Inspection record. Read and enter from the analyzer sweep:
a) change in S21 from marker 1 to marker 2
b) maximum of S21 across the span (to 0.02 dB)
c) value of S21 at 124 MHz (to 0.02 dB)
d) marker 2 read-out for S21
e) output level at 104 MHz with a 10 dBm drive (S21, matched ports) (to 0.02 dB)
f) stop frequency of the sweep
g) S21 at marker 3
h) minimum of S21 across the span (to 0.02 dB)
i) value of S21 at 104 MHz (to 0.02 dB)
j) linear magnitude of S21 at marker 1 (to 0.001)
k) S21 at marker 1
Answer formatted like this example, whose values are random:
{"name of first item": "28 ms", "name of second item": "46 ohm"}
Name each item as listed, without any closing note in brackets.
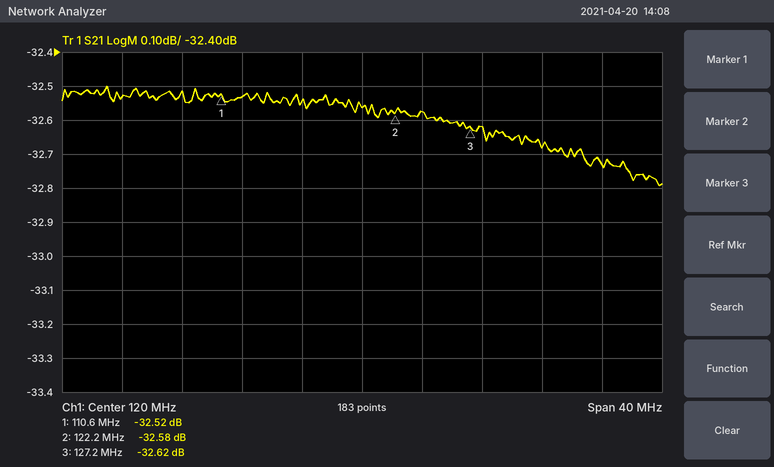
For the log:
{"change in S21 from marker 1 to marker 2": "-0.06 dB", "maximum of S21 across the span": "-32.50 dB", "value of S21 at 124 MHz": "-32.58 dB", "marker 2 read-out for S21": "-32.58 dB", "output level at 104 MHz with a 10 dBm drive (S21, matched ports)": "-22.54 dBm", "stop frequency of the sweep": "140 MHz", "S21 at marker 3": "-32.62 dB", "minimum of S21 across the span": "-32.80 dB", "value of S21 at 104 MHz": "-32.54 dB", "linear magnitude of S21 at marker 1": "0.024", "S21 at marker 1": "-32.52 dB"}
